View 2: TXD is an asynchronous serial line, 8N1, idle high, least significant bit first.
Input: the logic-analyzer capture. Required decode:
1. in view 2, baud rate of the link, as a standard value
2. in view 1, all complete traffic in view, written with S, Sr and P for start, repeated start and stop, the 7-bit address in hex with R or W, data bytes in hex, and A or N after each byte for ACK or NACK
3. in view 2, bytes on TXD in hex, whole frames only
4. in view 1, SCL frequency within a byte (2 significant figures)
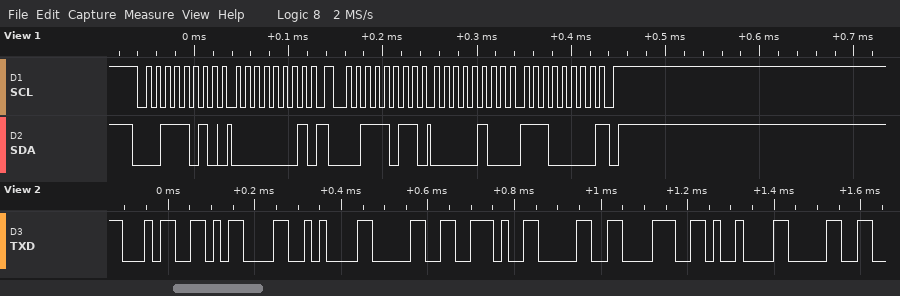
57600 baud
S 1DW A 01 A Sr 1DR A 04 A E0 N P
34 0D 0A 30 2E 30 38 09 30
100 kHz
